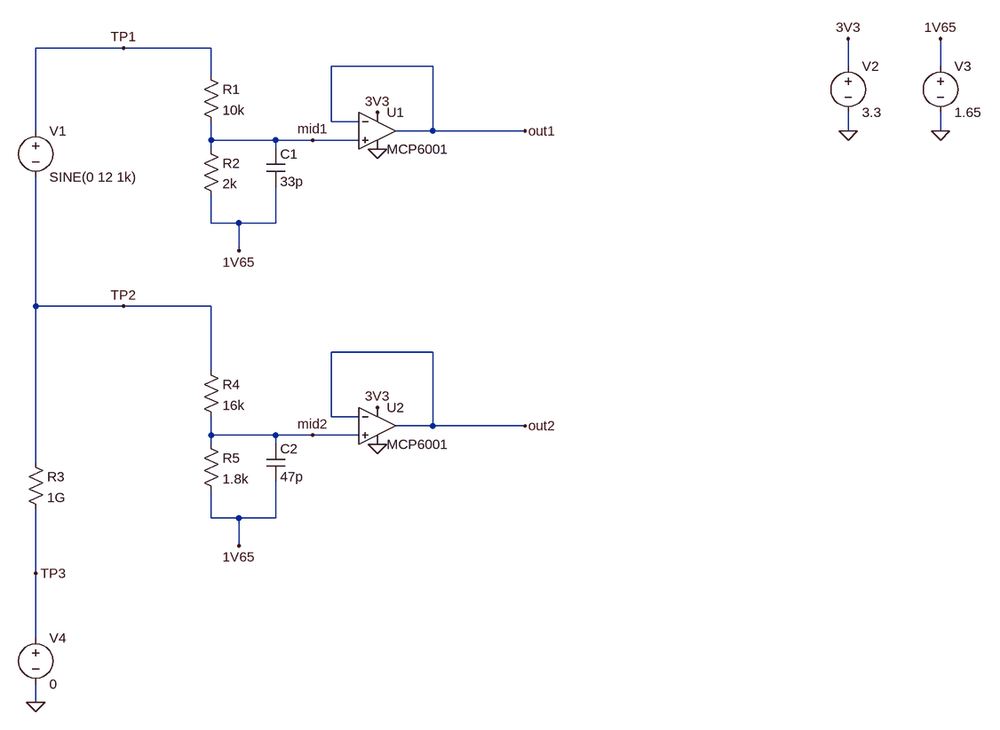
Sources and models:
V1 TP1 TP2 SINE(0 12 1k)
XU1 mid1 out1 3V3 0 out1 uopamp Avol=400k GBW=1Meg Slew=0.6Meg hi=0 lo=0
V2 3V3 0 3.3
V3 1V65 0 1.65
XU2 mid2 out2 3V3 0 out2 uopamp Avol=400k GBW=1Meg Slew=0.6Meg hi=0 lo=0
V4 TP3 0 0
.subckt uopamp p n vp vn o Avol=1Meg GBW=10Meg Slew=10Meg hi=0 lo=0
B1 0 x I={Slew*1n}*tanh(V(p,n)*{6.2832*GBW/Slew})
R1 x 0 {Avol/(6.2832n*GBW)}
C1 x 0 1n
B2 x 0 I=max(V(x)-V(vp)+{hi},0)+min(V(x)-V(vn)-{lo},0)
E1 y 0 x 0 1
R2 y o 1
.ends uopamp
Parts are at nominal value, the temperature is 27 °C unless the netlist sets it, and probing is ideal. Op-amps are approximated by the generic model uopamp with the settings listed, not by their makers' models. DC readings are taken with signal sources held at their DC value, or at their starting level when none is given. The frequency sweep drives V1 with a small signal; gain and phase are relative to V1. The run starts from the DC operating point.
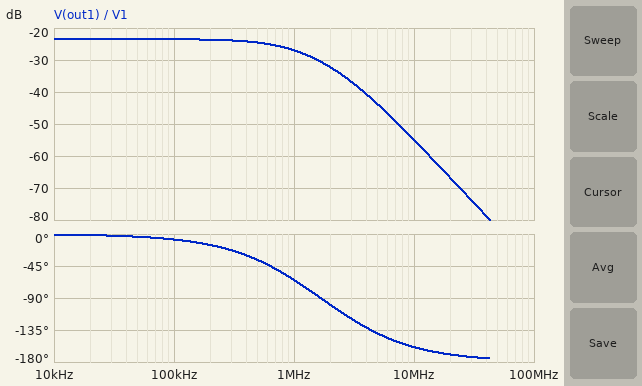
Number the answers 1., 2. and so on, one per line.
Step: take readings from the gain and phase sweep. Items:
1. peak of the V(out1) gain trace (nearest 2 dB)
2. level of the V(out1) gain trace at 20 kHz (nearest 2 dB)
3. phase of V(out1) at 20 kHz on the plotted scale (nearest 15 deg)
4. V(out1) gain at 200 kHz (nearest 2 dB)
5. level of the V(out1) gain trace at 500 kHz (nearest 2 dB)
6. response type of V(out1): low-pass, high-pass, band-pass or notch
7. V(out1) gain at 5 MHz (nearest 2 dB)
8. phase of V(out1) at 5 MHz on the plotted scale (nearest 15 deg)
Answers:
1. -24 dB
2. -24 dB
3. 0 deg
4. -24 dB
5. -24 dB
6. low-pass
7. -44 dB
8. -135 deg
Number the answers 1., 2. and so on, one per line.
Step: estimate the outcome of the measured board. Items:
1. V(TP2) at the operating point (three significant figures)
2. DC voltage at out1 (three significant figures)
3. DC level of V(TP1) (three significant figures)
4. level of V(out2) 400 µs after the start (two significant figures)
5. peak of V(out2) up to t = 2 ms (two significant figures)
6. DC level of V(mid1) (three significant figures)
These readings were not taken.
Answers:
1. 1.65 V
2. 1.65 V
3. 1.65 V
4. 1.2 V
5. 2.4 V
6. 1.65 V
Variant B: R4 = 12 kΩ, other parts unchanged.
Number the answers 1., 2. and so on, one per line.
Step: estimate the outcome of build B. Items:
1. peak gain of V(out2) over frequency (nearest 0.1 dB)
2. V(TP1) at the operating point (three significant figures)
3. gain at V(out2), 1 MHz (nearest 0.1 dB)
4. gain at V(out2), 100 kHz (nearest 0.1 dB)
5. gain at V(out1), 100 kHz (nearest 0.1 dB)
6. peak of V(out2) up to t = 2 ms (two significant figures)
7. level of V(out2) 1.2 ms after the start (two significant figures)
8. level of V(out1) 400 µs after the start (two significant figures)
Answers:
1. -23.1 dB
2. 1.65 V
3. -27.0 dB
4. -23.2 dB
5. -22.3 dB
6. 2.5 V
7. 850 mV
8. 2.2 V
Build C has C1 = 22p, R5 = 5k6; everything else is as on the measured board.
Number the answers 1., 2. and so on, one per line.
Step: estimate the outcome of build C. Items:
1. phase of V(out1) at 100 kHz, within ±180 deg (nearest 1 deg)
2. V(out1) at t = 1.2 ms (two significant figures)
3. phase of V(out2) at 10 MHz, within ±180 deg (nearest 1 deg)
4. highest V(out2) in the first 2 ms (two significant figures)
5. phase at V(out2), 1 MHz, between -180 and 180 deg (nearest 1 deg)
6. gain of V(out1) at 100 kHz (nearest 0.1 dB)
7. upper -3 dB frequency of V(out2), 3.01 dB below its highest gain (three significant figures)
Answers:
1. -6 deg
2. 2.3 V
3. 11 deg
4. 3.3 V
5. 82 deg
6. -24.5 dB
7. 539 kHz
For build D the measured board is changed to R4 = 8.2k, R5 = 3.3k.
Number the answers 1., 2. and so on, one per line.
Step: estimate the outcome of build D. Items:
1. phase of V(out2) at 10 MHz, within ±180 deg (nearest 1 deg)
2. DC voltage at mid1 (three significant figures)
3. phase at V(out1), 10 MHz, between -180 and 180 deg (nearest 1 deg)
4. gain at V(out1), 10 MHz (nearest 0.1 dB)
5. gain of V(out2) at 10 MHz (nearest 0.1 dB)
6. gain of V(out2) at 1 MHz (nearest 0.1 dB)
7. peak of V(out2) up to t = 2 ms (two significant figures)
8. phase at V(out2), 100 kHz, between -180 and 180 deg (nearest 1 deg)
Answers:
1. 14 deg
2. 1.65 V
3. -158 deg
4. -51.9 dB
5. -54.8 dB
6. -22.3 dB
7. 3.3 V
8. 170 deg
